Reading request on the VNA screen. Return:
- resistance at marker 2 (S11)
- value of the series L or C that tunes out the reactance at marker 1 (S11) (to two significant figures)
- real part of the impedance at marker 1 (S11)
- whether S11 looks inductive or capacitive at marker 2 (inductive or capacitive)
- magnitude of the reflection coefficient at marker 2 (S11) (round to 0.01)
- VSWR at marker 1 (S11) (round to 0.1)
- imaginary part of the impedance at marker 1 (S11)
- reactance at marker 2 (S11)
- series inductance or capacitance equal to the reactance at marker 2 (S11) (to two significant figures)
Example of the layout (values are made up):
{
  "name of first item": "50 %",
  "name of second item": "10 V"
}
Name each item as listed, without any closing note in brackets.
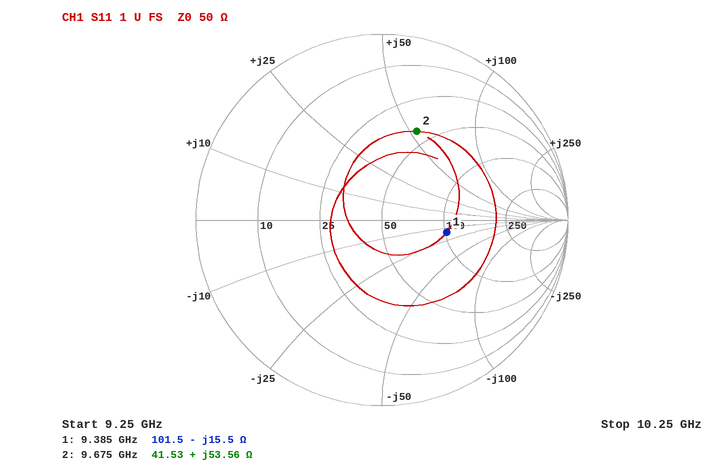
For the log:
{
  "resistance at marker 2": "41.53 Ω",
  "value of the series L or C that tunes out the reactance at marker 1 (S11)": "260 pH",
  "real part of the impedance at marker 1": "101.5 Ω",
  "whether S11 looks inductive or capacitive at marker 2": "inductive",
  "magnitude of the reflection coefficient at marker 2 (S11)": "0.51",
  "VSWR at marker 1 (S11)": "2.1",
  "imaginary part of the impedance at marker 1": "-15.5 Ω",
  "reactance at marker 2": "+53.56 Ω",
  "series inductance or capacitance equal to the reactance at marker 2 (S11)": "880 pH"
}
